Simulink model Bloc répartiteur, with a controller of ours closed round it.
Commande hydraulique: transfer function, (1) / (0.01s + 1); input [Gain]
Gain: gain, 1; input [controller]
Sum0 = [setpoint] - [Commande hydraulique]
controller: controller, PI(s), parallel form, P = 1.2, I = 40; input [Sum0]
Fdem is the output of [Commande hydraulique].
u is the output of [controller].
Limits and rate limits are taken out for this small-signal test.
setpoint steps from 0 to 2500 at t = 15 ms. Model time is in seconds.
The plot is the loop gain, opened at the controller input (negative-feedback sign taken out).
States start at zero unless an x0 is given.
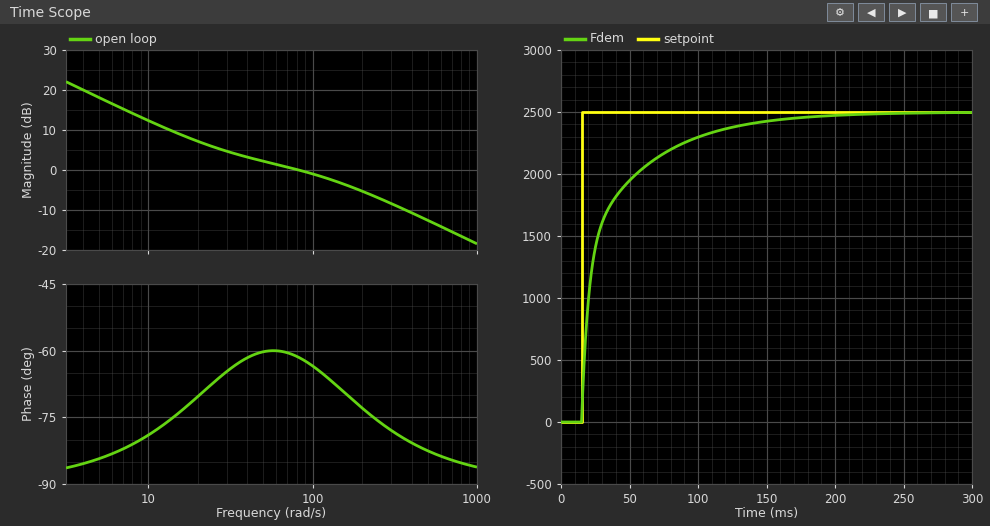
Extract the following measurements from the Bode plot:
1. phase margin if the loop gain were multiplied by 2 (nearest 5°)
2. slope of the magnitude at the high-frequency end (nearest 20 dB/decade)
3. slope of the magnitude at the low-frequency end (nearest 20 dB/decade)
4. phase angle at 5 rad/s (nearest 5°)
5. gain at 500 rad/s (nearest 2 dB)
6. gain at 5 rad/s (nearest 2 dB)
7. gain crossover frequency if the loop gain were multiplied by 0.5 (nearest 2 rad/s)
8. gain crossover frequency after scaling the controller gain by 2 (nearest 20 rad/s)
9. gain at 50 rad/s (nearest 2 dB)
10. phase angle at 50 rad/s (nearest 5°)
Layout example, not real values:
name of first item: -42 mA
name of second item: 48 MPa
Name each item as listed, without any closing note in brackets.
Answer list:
phase margin if the loop gain were multiplied by 2: 105°
slope of the magnitude at the high-frequency end: -20 dB/decade
slope of the magnitude at the low-frequency end: -20 dB/decade
phase angle at 5 rad/s: -85°
gain at 500 rad/s: -12 dB
gain at 5 rad/s: 18 dB
gain crossover frequency if the loop gain were multiplied by 0.5: 24 rad/s
gain crossover frequency after scaling the controller gain by 2: 220 rad/s
gain at 50 rad/s: 2 dB
phase angle at 50 rad/s: -60°
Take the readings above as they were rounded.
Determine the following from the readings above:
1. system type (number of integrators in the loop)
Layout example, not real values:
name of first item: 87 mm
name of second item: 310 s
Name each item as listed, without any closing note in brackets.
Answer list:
system type: 1
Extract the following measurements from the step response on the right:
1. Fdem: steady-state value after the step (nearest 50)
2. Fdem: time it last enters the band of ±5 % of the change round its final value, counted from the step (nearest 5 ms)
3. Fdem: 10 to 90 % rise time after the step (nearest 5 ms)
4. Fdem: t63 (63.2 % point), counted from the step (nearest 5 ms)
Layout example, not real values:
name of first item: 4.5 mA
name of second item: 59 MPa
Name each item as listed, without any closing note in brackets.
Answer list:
Fdem: steady-state value after the step: 2500
Fdem: time it last enters the band of ±5 % of the change round its final value, counted from the step: 110 ms
Fdem: 10 to 90 % rise time after the step: 75 ms
Fdem: t63 (63.2 % point), counted from the step: 15 ms
